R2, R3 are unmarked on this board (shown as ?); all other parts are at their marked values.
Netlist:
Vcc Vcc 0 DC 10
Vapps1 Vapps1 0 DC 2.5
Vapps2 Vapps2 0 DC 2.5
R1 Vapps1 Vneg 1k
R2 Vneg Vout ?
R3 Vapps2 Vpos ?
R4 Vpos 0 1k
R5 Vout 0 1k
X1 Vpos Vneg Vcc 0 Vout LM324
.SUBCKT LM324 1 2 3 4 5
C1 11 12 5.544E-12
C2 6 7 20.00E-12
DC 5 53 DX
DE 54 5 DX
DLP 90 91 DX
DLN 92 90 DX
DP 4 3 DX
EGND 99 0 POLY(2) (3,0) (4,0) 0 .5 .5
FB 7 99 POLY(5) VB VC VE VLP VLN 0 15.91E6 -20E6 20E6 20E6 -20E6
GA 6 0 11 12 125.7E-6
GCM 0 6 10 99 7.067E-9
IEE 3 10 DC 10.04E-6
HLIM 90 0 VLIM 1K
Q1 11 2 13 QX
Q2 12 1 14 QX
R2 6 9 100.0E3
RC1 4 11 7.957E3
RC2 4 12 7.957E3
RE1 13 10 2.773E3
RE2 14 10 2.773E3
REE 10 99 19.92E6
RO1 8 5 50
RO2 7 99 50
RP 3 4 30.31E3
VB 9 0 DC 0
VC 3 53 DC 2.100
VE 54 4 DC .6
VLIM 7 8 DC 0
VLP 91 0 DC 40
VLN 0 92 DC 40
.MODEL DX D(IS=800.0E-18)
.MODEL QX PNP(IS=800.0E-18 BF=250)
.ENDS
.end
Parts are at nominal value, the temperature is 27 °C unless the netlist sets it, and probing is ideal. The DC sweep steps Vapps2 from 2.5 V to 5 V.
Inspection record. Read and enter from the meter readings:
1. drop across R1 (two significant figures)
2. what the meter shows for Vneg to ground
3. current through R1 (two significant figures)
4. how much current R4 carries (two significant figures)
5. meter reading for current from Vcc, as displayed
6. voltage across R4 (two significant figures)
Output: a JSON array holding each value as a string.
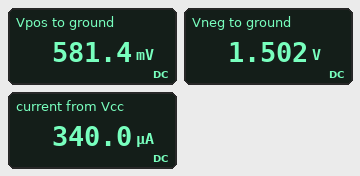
["1.0 V", "1.502 V", "1.0 mA", "580 µA", "340.0 µA", "580 mV"]
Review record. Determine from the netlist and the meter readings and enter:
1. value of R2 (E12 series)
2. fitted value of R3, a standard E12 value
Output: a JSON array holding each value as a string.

["1.5 kΩ", "3.3 kΩ"]
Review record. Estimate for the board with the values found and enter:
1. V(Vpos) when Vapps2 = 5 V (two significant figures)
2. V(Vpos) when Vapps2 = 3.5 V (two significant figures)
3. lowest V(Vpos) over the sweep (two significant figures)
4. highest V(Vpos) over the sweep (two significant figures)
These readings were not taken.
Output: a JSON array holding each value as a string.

["1.2 V", "810 mV", "580 mV", "1.2 V"]
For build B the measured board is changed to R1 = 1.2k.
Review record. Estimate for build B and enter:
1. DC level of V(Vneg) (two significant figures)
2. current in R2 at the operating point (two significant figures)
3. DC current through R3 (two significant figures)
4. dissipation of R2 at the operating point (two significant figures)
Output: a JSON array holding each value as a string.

["1.4 V", "920 µA", "580 µA", "1.3 mW"]
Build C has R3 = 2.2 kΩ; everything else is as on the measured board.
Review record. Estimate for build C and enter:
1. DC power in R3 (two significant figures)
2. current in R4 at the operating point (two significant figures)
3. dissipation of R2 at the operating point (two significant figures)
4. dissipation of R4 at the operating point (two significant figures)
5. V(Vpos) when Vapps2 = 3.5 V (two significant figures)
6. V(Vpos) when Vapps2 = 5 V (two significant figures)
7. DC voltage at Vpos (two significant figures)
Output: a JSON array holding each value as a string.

["1.3 mW", "780 µA", "1.5 mW", "610 µW", "1.1 V", "1.6 V", "780 mV"]
